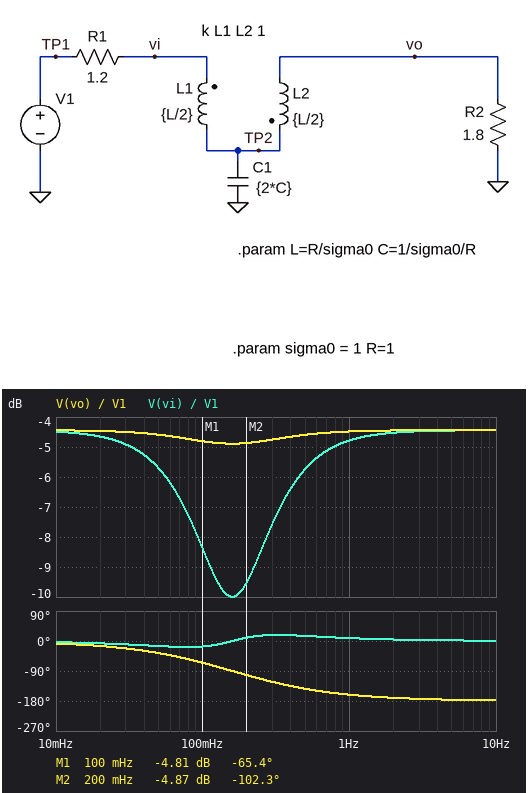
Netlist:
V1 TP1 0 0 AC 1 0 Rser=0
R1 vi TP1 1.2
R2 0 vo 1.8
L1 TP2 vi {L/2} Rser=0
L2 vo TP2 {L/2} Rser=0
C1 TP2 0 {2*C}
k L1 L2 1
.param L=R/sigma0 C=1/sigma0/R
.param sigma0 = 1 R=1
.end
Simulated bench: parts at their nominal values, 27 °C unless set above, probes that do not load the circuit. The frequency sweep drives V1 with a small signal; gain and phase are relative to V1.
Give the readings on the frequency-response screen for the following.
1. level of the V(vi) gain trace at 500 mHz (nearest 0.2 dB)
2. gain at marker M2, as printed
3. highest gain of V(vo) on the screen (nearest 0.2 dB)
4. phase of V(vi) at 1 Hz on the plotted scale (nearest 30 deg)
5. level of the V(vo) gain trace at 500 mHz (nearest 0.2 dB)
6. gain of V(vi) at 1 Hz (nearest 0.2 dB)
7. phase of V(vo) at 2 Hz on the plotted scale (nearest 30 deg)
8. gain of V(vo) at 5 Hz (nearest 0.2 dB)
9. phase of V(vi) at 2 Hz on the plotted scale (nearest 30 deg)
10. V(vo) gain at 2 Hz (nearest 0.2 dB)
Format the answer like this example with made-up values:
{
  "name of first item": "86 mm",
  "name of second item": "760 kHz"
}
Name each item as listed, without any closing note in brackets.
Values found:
{
  "level of the V(vi) gain trace at 500 mHz": "-5.8 dB",
  "gain at marker M2, as printed": "-4.87 dB",
  "highest gain of V(vo) on the screen": "-4.4 dB",
  "phase of V(vi) at 1 Hz on the plotted scale": "0 deg",
  "level of the V(vo) gain trace at 500 mHz": "-4.6 dB",
  "gain of V(vi) at 1 Hz": "-4.8 dB",
  "phase of V(vo) at 2 Hz on the plotted scale": "-180 deg",
  "gain of V(vo) at 5 Hz": "-4.4 dB",
  "phase of V(vi) at 2 Hz on the plotted scale": "0 deg",
  "V(vo) gain at 2 Hz": "-4.4 dB"
}
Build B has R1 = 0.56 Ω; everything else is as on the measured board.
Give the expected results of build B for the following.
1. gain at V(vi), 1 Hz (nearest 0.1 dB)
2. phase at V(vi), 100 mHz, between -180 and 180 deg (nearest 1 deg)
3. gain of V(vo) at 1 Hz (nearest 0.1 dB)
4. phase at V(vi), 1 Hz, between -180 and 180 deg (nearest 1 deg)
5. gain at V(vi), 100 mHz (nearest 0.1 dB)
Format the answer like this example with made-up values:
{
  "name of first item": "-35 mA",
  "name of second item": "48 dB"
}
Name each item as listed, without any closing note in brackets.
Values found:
{
  "gain at V(vi), 1 Hz": "-2.5 dB",
  "phase at V(vi), 100 mHz, between -180 and 180 deg": "-11 deg",
  "gain of V(vo) at 1 Hz": "-2.2 dB",
  "phase at V(vi), 1 Hz, between -180 and 180 deg": "5 deg",
  "gain at V(vi), 100 mHz": "-4.8 dB"
}
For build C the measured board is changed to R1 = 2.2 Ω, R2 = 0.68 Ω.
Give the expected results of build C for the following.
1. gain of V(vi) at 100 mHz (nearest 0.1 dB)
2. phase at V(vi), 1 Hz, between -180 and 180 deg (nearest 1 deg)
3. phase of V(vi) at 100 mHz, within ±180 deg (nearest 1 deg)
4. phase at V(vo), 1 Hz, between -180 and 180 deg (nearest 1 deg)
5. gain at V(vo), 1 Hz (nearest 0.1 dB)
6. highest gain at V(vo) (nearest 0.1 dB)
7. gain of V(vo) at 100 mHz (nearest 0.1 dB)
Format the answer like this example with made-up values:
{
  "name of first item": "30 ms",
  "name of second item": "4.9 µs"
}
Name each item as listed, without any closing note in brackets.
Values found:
{
  "gain of V(vi) at 100 mHz": "-8.7 dB",
  "phase at V(vi), 1 Hz, between -180 and 180 deg": "-10 deg",
  "phase of V(vi) at 100 mHz, within ±180 deg": "11 deg",
  "phase at V(vo), 1 Hz, between -180 and 180 deg": "-164 deg",
  "gain at V(vo), 1 Hz": "-12.4 dB",
  "highest gain at V(vo)": "-11.3 dB",
  "gain of V(vo) at 100 mHz": "-11.6 dB"
}
